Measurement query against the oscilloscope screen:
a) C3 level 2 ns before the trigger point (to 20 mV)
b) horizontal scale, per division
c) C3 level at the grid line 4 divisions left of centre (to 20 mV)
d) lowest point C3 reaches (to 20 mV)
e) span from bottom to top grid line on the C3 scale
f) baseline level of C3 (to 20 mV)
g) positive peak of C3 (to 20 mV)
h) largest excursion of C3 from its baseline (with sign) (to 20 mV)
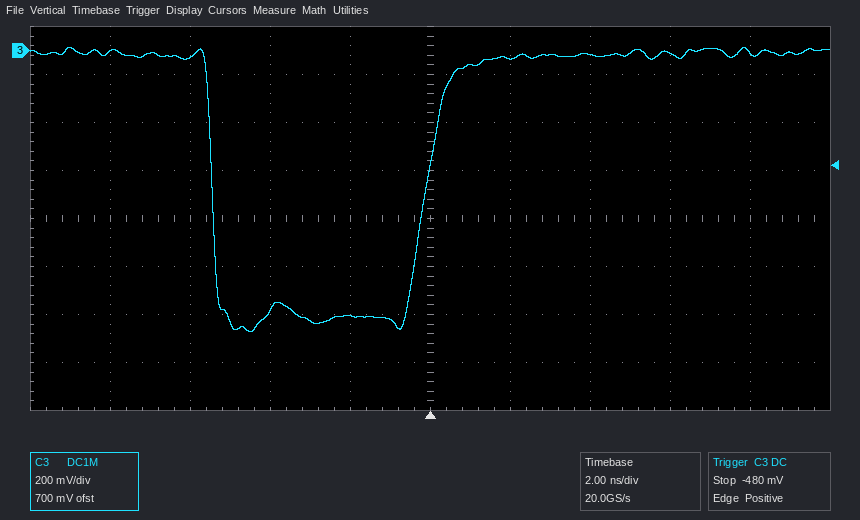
-1.10 V
2 ns
0 mV
-1.18 V
1.6 V
-20 mV
20 mV
-1.16 V
